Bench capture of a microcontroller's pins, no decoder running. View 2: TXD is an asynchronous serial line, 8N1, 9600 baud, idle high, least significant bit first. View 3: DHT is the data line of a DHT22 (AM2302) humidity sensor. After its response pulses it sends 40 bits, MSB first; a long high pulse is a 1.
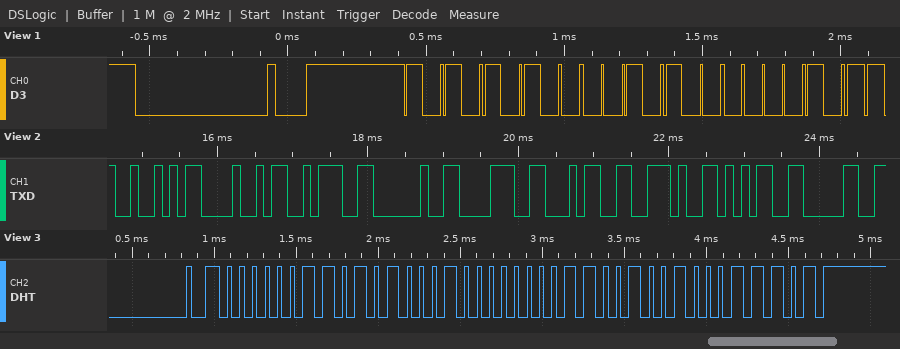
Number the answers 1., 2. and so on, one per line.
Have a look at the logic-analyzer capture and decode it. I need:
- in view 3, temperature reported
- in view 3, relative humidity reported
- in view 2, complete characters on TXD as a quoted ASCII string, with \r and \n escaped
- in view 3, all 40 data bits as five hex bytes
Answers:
1. 20.1 °C
2. 84.9 %
3. "RH: 84.50"
4. 03 51 00 C9 1D
